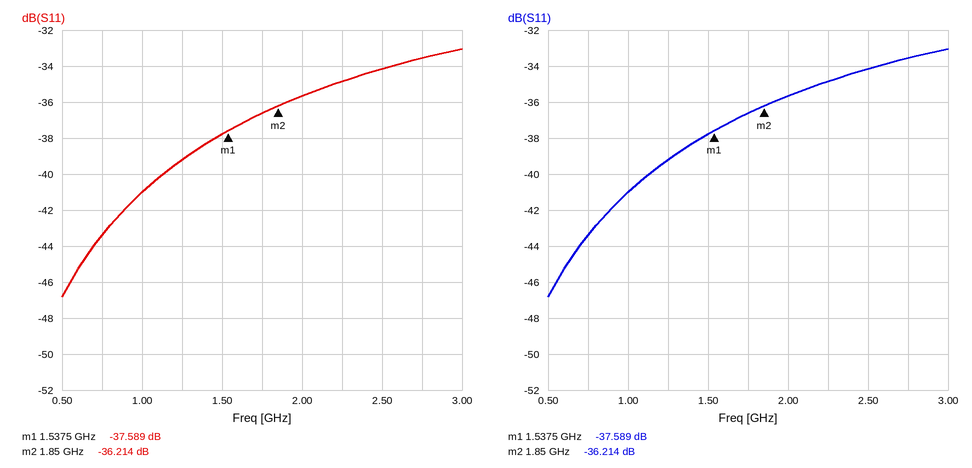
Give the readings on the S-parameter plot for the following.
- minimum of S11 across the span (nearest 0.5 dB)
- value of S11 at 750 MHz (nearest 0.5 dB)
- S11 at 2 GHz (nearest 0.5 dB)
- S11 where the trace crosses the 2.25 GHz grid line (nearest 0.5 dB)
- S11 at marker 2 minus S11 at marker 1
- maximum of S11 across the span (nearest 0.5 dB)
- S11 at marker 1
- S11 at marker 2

-47.0 dB
-43.5 dB
-35.5 dB
-35.0 dB
1.375 dB
-33.0 dB
-37.589 dB
-36.214 dB
